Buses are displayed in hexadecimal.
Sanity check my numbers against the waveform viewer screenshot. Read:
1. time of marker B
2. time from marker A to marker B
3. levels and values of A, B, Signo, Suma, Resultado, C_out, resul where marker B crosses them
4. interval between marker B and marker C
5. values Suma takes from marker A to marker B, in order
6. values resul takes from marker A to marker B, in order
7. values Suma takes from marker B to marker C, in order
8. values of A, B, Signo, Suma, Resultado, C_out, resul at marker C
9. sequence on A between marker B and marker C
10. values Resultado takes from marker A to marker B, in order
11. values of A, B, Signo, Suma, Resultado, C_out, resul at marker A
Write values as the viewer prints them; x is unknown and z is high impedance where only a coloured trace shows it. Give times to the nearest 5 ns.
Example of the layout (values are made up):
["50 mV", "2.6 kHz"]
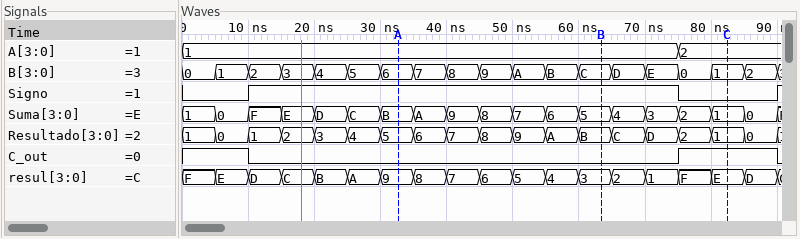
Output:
["65 ns", "30 ns", "A=1, B=C, Signo=1, Suma=5, Resultado=B, C_out=0, resul=3", "20 ns", "B, A, 9, 8, 7, 6, 5", "9, 8, 7, 6, 5, 4, 3", "5, 4, 3, 2, 1", "A=2, B=1, Signo=0, Suma=1, Resultado=1, C_out=1, resul=E", "1, 2", "5, 6, 7, 8, 9, A, B", "A=1, B=6, Signo=1, Suma=B, Resultado=5, C_out=0, resul=9"]
